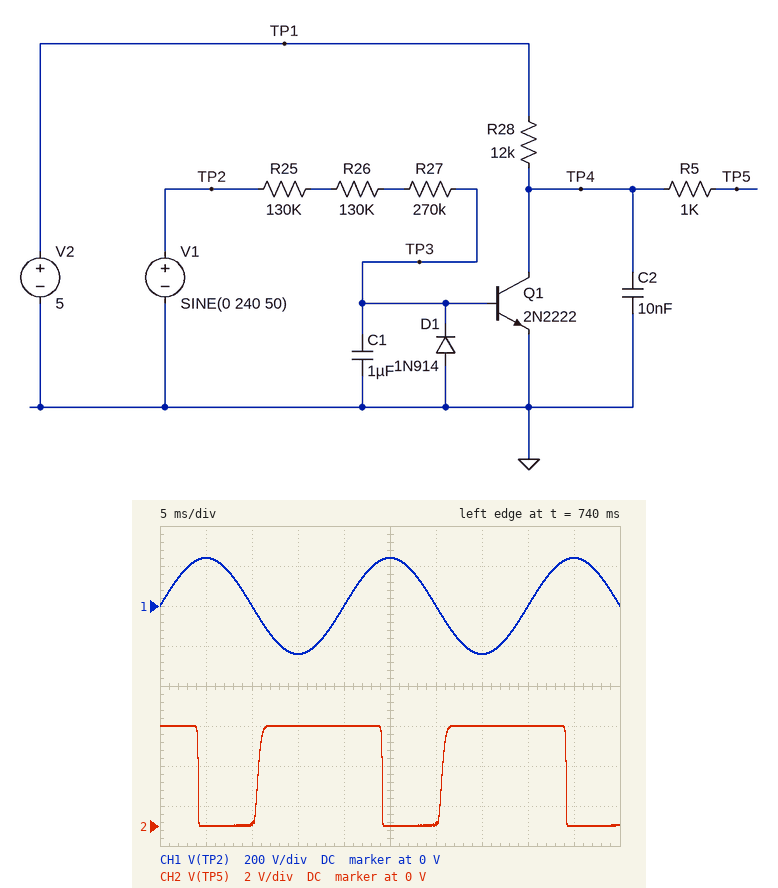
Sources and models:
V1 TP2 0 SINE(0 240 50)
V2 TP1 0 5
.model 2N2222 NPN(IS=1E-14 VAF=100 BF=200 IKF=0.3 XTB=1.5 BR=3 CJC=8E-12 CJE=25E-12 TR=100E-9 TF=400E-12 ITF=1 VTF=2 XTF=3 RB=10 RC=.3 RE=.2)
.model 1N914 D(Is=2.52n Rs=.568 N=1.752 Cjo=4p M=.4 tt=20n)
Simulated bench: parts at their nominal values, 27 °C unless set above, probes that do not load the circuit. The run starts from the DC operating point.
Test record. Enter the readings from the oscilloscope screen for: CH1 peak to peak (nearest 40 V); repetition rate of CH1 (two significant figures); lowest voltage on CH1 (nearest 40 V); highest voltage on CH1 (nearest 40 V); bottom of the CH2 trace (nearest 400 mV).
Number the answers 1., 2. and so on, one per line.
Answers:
1. 480 V
2. 50 Hz
3. -240 V
4. 240 V
5. 0 V
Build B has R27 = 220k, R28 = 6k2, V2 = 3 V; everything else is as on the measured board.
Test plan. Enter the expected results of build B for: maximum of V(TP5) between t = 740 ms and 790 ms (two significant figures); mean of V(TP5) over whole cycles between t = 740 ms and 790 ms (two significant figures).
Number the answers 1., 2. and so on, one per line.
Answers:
1. 3.0 V
2. 2.0 V
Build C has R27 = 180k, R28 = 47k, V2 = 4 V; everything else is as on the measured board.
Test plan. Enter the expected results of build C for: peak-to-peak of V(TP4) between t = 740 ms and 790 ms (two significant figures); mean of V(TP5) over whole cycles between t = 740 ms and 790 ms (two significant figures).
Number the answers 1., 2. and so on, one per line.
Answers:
1. 4.0 V
2. 2.5 V
